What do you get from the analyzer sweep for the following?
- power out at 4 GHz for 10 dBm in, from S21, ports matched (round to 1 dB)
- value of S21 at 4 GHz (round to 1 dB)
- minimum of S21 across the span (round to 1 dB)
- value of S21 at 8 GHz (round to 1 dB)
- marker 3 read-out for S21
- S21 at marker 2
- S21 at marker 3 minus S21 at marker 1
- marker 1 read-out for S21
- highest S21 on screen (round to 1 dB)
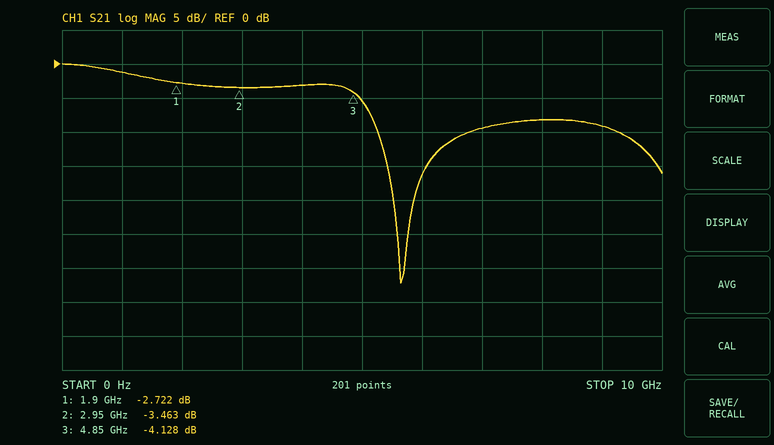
7 dBm
-3 dB
-32 dB
-8 dB
-4.128 dB
-3.463 dB
-1.406 dB
-2.722 dB
0 dB
